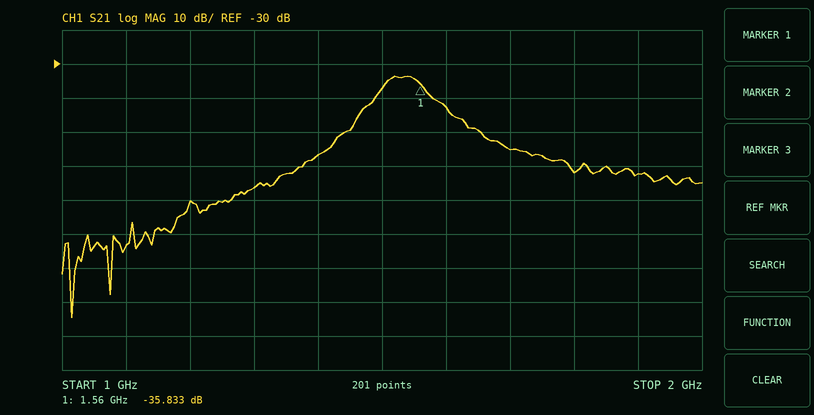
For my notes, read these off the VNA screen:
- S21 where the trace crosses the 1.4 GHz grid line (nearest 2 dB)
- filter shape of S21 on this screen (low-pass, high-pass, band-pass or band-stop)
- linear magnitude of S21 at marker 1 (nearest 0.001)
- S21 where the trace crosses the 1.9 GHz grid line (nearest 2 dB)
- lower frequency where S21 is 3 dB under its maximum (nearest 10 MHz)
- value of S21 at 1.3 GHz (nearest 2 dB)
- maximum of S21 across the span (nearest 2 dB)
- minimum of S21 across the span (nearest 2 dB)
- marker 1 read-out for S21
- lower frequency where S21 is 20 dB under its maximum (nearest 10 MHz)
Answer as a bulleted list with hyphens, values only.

- -56 dB
- band-pass
- 0.016
- -62 dB
- 1.50 GHz
- -66 dB
- -34 dB
- -104 dB
- -35.833 dB
- 1.42 GHz
